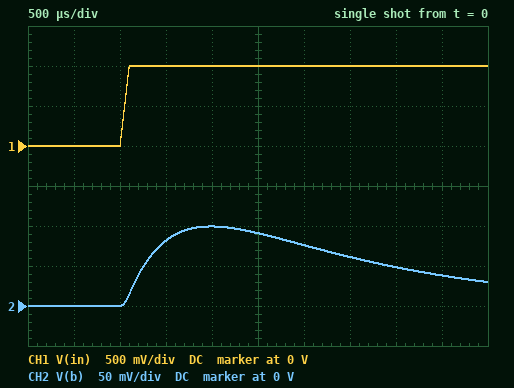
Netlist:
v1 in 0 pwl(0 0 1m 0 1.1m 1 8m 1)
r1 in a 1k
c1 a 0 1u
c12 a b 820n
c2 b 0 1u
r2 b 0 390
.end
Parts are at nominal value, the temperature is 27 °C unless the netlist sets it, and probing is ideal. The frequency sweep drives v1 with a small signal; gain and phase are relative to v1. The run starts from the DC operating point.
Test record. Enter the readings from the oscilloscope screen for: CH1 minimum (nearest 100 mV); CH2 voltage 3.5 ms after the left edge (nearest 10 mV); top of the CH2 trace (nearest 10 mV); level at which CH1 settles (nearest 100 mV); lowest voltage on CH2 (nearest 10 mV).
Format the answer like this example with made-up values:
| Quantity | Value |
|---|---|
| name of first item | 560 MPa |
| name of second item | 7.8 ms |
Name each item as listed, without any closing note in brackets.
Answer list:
| Quantity | Value |
|---|---|
| CH1 minimum | 0 V |
| CH2 voltage 3.5 ms after the left edge | 60 mV |
| top of the CH2 trace | 100 mV |
| level at which CH1 settles | 1.0 V |
| lowest voltage on CH2 | 0 V |
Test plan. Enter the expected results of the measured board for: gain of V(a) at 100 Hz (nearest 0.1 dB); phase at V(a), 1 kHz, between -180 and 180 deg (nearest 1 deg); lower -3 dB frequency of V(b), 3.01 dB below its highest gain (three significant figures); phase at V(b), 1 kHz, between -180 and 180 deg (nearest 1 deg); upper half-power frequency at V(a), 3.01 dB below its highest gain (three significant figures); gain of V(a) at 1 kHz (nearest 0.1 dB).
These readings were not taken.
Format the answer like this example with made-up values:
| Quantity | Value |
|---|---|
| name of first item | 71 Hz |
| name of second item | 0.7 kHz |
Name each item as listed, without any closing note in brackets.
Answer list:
| Quantity | Value |
|---|---|
| gain of V(a) at 100 Hz | -3.8 dB |
| phase at V(a), 1 kHz, between -180 and 180 deg | -81 deg |
| lower -3 dB frequency of V(b), 3.01 dB below its highest gain | 55.1 Hz |
| phase at V(b), 1 kHz, between -180 and 180 deg | -68 deg |
| upper half-power frequency at V(a), 3.01 dB below its highest gain | 83.6 Hz |
| gain of V(a) at 1 kHz | -19.4 dB |
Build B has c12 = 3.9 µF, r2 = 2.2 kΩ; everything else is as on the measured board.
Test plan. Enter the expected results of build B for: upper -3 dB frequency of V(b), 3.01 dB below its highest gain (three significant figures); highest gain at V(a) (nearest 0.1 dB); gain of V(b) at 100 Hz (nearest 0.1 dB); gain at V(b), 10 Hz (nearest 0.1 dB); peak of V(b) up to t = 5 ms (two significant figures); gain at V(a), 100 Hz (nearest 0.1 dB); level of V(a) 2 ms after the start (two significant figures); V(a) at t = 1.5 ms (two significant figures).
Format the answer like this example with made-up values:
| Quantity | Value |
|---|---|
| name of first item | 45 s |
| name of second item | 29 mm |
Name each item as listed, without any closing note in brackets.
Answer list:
| Quantity | Value |
|---|---|
| upper -3 dB frequency of V(b), 3.01 dB below its highest gain | 138 Hz |
| highest gain at V(a) | 0 dB |
| gain of V(b) at 100 Hz | -6.9 dB |
| gain at V(b), 10 Hz | -8.0 dB |
| peak of V(b) up to t = 5 ms | 470 mV |
| gain at V(a), 100 Hz | -4.8 dB |
| level of V(a) 2 ms after the start | 380 mV |
| V(a) at t = 1.5 ms | 210 mV |
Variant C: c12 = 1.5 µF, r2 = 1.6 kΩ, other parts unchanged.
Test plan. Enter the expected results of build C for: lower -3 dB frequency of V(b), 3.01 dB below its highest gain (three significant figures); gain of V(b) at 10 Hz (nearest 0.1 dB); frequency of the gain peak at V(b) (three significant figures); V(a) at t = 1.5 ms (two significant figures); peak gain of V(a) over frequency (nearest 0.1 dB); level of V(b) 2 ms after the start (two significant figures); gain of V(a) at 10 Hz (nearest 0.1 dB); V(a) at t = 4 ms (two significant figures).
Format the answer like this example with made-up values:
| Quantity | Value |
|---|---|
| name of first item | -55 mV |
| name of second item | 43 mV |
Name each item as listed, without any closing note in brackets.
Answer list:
| Quantity | Value |
|---|---|
| lower -3 dB frequency of V(b), 3.01 dB below its highest gain | 21.6 Hz |
| gain of V(b) at 10 Hz | -16.9 dB |
| frequency of the gain peak at V(b) | 62.9 Hz |
| V(a) at t = 1.5 ms | 240 mV |
| peak gain of V(a) over frequency | 0 dB |
| level of V(b) 2 ms after the start | 220 mV |
| gain of V(a) at 10 Hz | -0.2 dB |
| V(a) at t = 4 ms | 760 mV |
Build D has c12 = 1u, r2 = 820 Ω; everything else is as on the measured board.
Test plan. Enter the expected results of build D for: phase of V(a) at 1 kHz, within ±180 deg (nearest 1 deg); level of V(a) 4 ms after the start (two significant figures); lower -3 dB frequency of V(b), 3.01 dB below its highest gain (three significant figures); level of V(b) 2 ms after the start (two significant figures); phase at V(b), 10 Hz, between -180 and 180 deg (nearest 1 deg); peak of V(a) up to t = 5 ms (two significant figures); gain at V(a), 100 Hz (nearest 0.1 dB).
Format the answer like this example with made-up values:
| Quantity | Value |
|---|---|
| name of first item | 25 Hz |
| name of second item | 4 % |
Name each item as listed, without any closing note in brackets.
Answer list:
| Quantity | Value |
|---|---|
| phase of V(a) at 1 kHz, within ±180 deg | -82 deg |
| level of V(a) 4 ms after the start | 780 mV |
| lower -3 dB frequency of V(b), 3.01 dB below its highest gain | 37.7 Hz |
| level of V(b) 2 ms after the start | 160 mV |
| phase at V(b), 10 Hz, between -180 and 180 deg | 77 deg |
| peak of V(a) up to t = 5 ms | 850 mV |
| gain at V(a), 100 Hz | -4.0 dB |
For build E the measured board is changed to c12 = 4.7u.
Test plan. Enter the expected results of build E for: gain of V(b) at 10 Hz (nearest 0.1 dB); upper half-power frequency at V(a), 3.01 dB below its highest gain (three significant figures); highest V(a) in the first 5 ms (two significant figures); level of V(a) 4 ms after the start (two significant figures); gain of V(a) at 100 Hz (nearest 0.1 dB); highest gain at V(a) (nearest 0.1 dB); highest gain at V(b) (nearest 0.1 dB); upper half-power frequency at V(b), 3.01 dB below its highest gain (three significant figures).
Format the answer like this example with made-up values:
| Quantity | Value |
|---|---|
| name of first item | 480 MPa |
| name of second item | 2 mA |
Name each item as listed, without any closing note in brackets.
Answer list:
| Quantity | Value |
|---|---|
| gain of V(b) at 10 Hz | -19.6 dB |
| upper half-power frequency at V(a), 3.01 dB below its highest gain | 23.7 Hz |
| highest V(a) in the first 5 ms | 560 mV |
| level of V(a) 4 ms after the start | 490 mV |
| gain of V(a) at 100 Hz | -9.3 dB |
| highest gain at V(a) | 0 dB |
| highest gain at V(b) | -12.7 dB |
| upper half-power frequency at V(b), 3.01 dB below its highest gain | 330 Hz |
